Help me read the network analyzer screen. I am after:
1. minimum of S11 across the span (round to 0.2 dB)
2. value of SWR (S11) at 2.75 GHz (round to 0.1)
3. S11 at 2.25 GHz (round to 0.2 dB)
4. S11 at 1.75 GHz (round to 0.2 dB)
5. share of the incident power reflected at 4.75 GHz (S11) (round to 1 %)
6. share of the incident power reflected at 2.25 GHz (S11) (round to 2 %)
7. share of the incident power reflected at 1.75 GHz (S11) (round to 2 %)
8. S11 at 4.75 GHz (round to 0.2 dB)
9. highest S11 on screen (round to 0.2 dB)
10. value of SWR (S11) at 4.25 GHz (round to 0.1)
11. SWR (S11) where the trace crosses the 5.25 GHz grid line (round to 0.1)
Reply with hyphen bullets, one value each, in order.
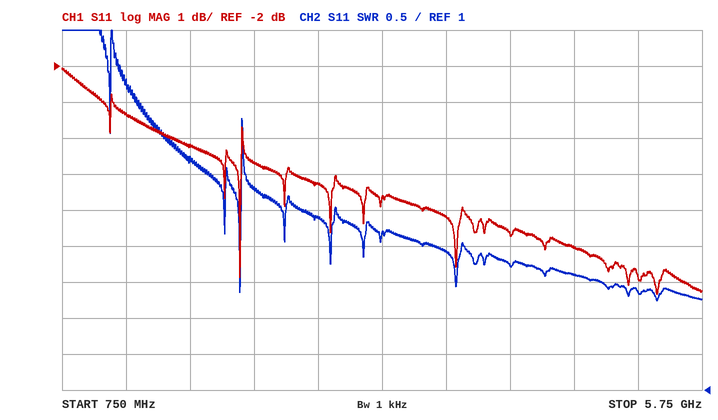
- -8.4 dB
- 3.4
- -4.6 dB
- -4.2 dB
- 20 %
- 34 %
- 38 %
- -7.0 dB
- -2.0 dB
- 2.7
- 2.4
